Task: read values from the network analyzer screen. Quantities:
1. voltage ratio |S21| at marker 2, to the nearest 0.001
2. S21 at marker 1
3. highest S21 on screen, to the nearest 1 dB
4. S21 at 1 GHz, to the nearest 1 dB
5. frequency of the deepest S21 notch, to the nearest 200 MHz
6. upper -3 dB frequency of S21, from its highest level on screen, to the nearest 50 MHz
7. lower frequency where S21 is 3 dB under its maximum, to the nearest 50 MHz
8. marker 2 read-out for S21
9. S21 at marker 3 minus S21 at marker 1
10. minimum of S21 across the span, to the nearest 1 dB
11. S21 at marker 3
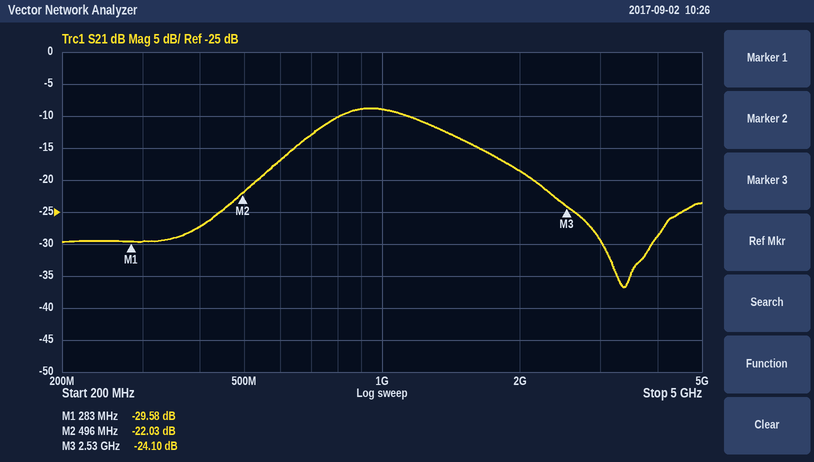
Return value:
0.079
-29.58 dB
-9 dB
-9 dB
3.4 GHz
1.30 GHz
750 MHz
-22.03 dB
5.48 dB
-37 dB
-24.10 dB
